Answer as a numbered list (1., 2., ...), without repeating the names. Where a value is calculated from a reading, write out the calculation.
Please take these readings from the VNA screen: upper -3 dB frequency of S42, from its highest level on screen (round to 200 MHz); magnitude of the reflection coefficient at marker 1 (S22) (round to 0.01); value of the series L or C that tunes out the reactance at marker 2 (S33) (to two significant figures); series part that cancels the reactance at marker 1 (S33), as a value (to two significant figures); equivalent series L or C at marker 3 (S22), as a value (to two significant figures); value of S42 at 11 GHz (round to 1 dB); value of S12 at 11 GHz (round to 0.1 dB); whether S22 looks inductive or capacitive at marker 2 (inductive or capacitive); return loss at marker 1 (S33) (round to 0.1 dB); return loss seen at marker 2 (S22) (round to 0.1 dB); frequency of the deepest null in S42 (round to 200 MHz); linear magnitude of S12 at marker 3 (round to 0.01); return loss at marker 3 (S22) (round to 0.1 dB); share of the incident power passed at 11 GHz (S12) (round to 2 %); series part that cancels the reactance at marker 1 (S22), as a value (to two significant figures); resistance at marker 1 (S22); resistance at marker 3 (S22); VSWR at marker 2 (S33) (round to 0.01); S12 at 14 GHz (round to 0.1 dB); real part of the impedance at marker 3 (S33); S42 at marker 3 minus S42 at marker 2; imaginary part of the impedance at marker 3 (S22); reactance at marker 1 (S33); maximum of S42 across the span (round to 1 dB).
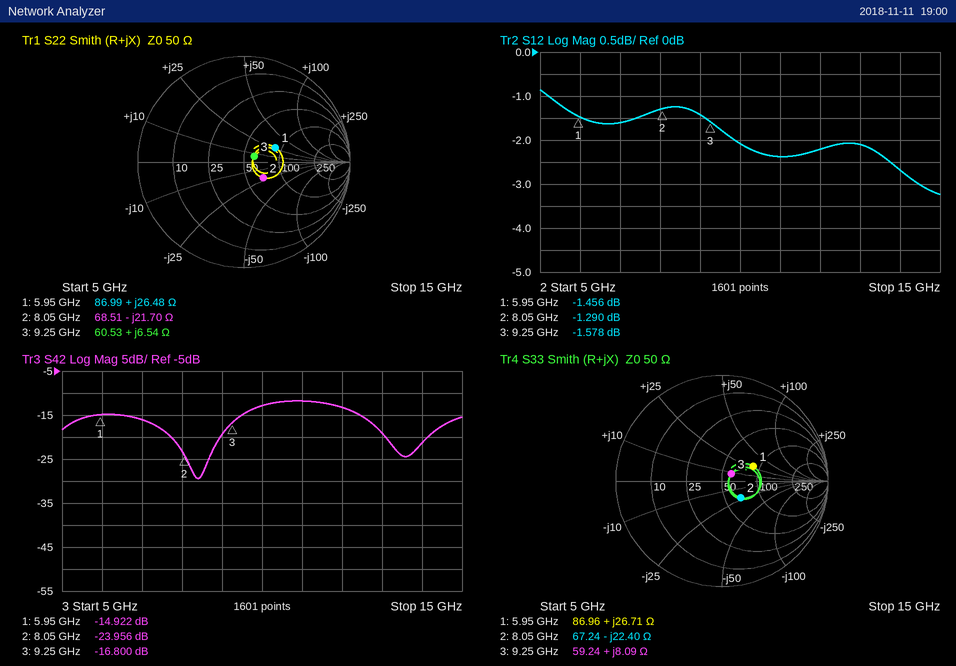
1. 12.4 GHz
2. 0.33
3. L = 22.4 Ω/(2π × 8.05 GHz) ≈ 443 pH, so 440 pH to two significant figures
4. C = 1/(2π × 5.95 GHz × 26.71 Ω) ≈ 1.0 pF
5. L = 6.54 Ω/(2π × 9.25 GHz) ≈ 113 pH, so 110 pH to two significant figures
6. -12 dB
7. -2.4 dB
8. capacitive
9. 9.7 dB
10. 12.5 dB
11. 8.4 GHz
12. 10^(-1.578/20) ≈ 0.83
13. 19.0 dB
14. 10^(-2.4/10) ≈ 58 %
15. C = 1/(2π × 5.95 GHz × 26.48 Ω) ≈ 1.0 pF
16. 86.99 Ω
17. 60.53 Ω
18. 1.62
19. -2.7 dB
20. 59.24 Ω
21. -16.8 − (-23.956) = 7.156 dB
22. +6.54 Ω
23. +26.71 Ω
24. -12 dB
